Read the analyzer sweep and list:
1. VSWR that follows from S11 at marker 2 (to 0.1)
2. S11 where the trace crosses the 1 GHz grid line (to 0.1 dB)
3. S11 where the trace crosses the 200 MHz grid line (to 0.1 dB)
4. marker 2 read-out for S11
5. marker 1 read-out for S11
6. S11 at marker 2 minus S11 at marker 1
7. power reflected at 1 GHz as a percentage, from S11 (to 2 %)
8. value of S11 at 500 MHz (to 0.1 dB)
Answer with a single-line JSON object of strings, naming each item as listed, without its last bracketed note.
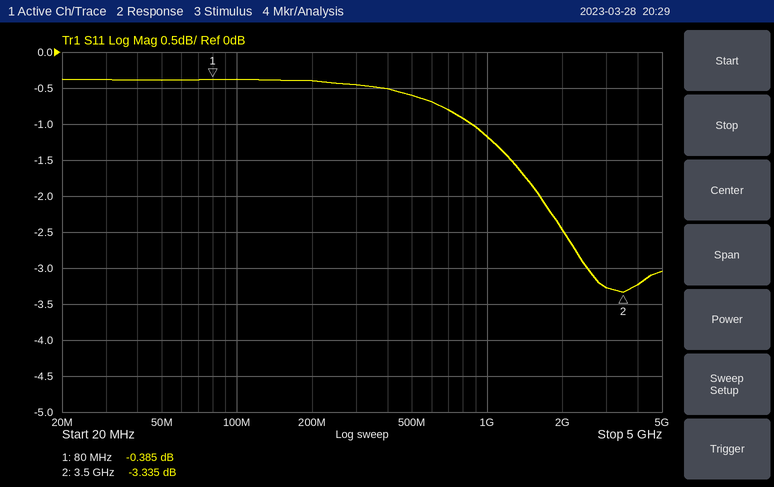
{"VSWR that follows from S11 at marker 2": "5.3", "S11 where the trace crosses the 1 GHz grid line": "-1.2 dB", "S11 where the trace crosses the 200 MHz grid line": "-0.4 dB", "marker 2 read-out for S11": "-3.335 dB", "marker 1 read-out for S11": "-0.385 dB", "S11 at marker 2 minus S11 at marker 1": "-2.950 dB", "power reflected at 1 GHz as a percentage, from S11": "76 %", "value of S11 at 500 MHz": "-0.6 dB"}
